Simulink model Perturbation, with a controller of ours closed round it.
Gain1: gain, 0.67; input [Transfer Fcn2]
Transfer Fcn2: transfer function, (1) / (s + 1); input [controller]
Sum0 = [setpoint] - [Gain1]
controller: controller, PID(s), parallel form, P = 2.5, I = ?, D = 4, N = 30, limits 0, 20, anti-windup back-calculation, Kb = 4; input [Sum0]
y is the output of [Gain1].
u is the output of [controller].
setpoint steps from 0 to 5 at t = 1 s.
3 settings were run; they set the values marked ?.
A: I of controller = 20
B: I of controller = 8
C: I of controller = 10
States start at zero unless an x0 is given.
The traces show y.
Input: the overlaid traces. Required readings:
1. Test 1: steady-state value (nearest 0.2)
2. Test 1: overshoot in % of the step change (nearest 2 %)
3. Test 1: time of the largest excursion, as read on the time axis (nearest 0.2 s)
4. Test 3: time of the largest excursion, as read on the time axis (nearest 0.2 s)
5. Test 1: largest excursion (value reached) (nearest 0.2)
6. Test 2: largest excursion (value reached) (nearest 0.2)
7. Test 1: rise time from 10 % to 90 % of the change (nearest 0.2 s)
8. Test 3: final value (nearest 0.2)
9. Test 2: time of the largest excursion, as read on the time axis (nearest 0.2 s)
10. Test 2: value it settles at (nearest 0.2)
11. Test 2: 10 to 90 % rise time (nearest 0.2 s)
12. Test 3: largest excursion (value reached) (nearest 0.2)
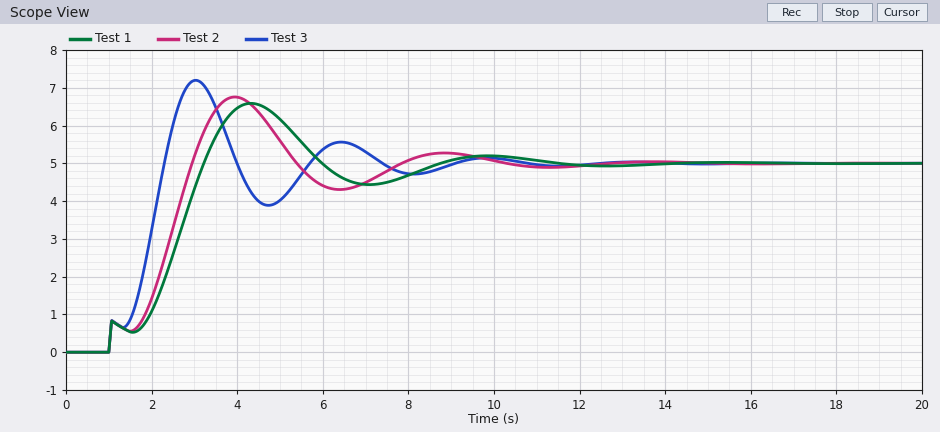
5.0
32 %
4.4 s
3.0 s
6.6
6.8
2.0 s
5.0
4.0 s
5.0
1.8 s
7.2
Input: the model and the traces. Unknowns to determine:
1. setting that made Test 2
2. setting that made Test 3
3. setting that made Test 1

C
A
B
